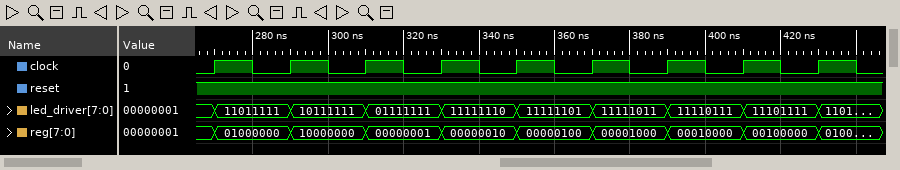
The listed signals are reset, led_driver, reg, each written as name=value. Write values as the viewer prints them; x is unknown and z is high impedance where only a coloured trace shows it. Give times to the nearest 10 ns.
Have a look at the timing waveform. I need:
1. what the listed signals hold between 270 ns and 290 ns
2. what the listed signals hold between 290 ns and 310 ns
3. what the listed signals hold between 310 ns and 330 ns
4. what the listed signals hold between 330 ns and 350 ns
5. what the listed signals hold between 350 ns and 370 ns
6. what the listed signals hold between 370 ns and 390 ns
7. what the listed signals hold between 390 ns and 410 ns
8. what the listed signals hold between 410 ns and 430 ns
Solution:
reset=1, led_driver=11011111, reg=01000000
reset=1, led_driver=10111111, reg=10000000
reset=1, led_driver=01111111, reg=00000001
reset=1, led_driver=11111110, reg=00000010
reset=1, led_driver=11111101, reg=00000100
reset=1, led_driver=11111011, reg=00001000
reset=1, led_driver=11110111, reg=00010000
reset=1, led_driver=11101111, reg=00100000
